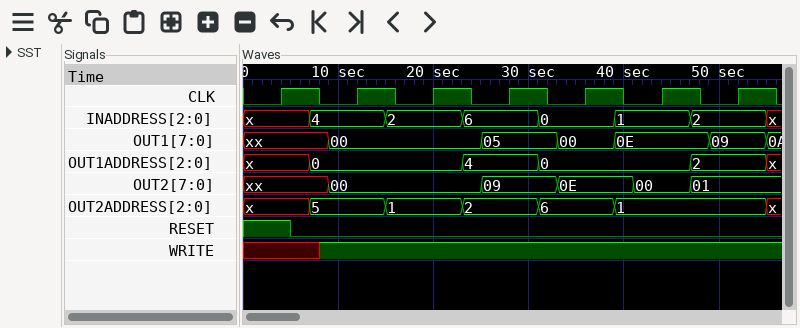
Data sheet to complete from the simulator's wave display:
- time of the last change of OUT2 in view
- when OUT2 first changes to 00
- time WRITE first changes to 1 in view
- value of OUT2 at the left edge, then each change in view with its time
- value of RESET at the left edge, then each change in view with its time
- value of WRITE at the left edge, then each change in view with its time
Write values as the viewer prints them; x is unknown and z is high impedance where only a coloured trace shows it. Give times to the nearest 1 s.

47 s
9 s
8 s
xx, 00 at 9 s, 09 at 25 s, 0E at 33 s, 00 at 41 s, 01 at 47 s
1, 0 at 5 s
x, 1 at 8 s
